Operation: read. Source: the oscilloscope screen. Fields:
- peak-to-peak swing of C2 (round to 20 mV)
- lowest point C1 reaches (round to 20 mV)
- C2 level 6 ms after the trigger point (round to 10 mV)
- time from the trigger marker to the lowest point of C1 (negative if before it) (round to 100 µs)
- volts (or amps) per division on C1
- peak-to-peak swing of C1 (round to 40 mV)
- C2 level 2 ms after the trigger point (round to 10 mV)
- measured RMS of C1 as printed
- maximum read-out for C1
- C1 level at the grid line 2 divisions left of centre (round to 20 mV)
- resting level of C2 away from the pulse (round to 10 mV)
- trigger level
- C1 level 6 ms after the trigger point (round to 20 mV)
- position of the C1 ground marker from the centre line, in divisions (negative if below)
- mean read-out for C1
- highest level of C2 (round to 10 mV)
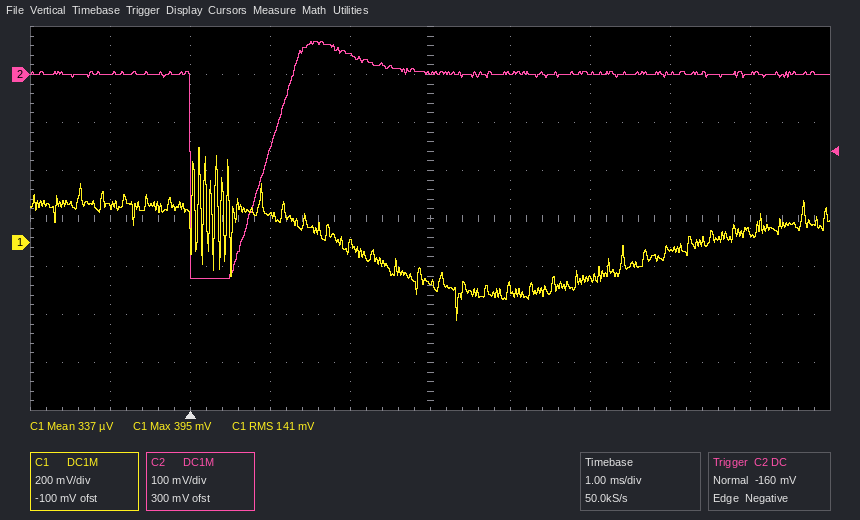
500 mV
-320 mV
0 mV
+3.3 ms
200 mV
720 mV
40 mV
141 mV
395 mV
120 mV
0 mV
-160 mV
-20 mV
-0.5 div
337 µV
70 mV
